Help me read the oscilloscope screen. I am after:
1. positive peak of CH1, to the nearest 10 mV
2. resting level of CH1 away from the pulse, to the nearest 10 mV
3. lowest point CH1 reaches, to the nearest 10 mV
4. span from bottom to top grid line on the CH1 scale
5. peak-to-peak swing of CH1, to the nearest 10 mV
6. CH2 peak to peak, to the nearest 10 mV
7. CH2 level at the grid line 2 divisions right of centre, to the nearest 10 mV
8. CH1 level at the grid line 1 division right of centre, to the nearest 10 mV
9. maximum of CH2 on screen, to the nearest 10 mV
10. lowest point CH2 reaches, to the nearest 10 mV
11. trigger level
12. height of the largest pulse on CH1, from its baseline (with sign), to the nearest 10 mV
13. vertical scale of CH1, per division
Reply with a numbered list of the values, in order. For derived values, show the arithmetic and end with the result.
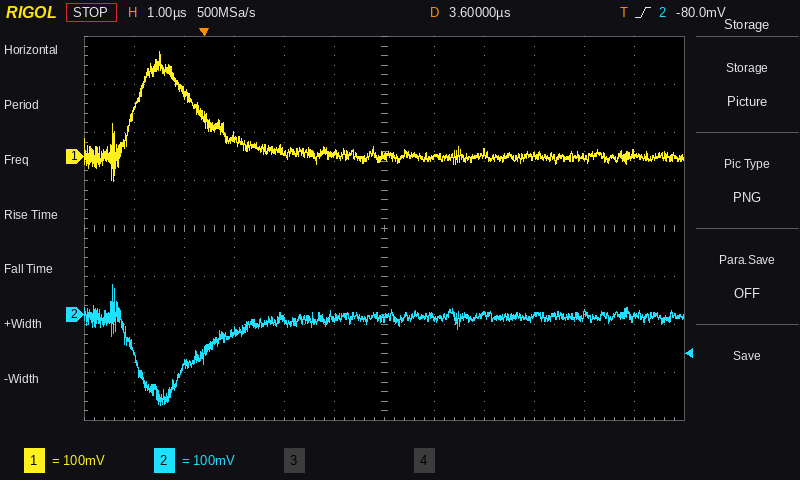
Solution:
1. 220 mV
2. 0 mV
3. -50 mV
4. 800 mV
5. 220 mV − (-50 mV) = 270 mV
6. 60 mV − (-190 mV) = 250 mV
7. 0 mV
8. 0 mV
9. 60 mV
10. -190 mV
11. -80.0 mV
12. 220 mV − (0 mV) = +220 mV
13. 100 mV
